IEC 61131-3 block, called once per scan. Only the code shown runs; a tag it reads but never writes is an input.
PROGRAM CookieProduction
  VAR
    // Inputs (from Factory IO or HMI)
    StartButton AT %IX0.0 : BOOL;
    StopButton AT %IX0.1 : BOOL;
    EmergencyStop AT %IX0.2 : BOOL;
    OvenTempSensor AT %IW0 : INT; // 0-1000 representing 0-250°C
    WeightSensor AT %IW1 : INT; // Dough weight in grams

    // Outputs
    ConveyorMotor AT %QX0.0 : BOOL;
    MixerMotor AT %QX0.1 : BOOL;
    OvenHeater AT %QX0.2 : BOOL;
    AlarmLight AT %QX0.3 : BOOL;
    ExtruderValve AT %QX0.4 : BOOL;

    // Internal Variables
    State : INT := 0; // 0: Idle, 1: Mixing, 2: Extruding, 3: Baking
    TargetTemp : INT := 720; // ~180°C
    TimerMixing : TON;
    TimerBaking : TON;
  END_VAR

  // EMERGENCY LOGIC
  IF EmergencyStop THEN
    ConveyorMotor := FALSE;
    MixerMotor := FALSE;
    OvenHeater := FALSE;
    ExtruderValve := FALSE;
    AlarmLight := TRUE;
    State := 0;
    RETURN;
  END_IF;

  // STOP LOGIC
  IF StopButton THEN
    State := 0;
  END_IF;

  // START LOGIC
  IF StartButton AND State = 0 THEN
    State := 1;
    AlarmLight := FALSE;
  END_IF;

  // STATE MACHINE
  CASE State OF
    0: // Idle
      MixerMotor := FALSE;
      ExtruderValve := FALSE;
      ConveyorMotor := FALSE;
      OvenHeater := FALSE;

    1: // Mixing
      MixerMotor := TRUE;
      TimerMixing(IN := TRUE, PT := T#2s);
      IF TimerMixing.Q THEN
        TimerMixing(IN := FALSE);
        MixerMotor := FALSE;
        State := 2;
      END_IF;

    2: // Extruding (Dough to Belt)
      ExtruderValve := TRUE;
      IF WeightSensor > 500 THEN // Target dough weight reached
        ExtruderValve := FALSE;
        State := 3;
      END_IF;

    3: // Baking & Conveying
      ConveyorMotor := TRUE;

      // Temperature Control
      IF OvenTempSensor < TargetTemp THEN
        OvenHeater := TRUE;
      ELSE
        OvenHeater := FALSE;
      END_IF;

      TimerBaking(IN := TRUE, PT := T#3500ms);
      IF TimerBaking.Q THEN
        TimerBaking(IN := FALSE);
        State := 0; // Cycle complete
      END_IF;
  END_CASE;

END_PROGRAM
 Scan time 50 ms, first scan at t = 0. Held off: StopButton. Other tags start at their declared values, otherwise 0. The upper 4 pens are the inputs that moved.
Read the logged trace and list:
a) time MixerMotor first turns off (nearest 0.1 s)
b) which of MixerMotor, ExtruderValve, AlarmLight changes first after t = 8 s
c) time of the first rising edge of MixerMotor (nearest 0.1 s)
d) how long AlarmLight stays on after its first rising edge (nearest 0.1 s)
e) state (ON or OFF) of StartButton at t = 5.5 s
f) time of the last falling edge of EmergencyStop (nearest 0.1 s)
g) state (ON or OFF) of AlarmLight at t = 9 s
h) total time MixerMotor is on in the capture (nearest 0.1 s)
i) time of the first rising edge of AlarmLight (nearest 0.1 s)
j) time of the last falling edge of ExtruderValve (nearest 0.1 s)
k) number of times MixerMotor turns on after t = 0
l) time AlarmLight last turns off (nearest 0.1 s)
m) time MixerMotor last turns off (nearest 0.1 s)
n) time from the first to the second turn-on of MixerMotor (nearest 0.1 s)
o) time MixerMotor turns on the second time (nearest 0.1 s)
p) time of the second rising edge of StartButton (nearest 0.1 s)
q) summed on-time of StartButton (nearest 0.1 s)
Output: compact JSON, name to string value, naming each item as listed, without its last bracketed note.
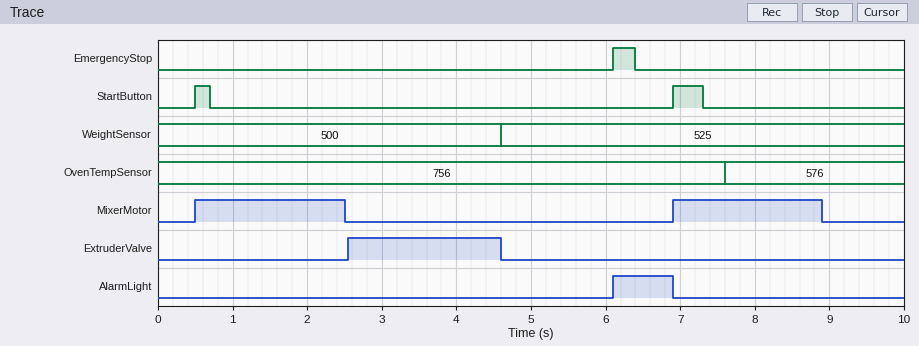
{"time MixerMotor first turns off": "2.5 s", "which of MixerMotor, ExtruderValve, AlarmLight changes first after t = 8 s": "MixerMotor", "time of the first rising edge of MixerMotor": "0.5 s", "how long AlarmLight stays on after its first rising edge": "0.8 s", "state (ON or OFF) of StartButton at t = 5.5 s": "OFF", "time of the last falling edge of EmergencyStop": "6.4 s", "state (ON or OFF) of AlarmLight at t = 9 s": "OFF", "total time MixerMotor is on in the capture": "4.0 s", "time of the first rising edge of AlarmLight": "6.1 s", "time of the last falling edge of ExtruderValve": "4.6 s", "number of times MixerMotor turns on after t = 0": "2", "time AlarmLight last turns off": "6.9 s", "time MixerMotor last turns off": "8.9 s", "time from the first to the second turn-on of MixerMotor": "6.4 s", "time MixerMotor turns on the second time": "6.9 s", "time of the second rising edge of StartButton": "6.9 s", "summed on-time of StartButton": "0.6 s"}
